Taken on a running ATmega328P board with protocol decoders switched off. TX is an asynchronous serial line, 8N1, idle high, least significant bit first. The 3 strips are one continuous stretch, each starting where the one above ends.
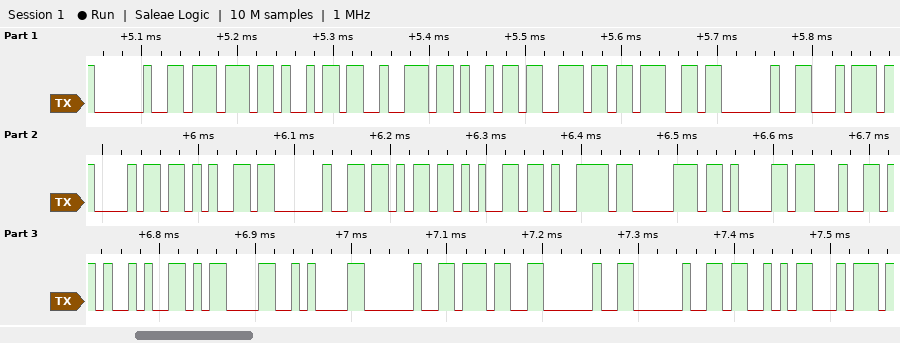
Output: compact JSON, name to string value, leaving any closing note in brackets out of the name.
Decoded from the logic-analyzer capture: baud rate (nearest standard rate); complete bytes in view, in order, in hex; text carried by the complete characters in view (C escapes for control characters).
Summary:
{"baud rate": "115200 baud", "complete bytes in view, in order, in hex": "20 77 69 72 69 6E 67 20 74 68 65 20 6B 65 79 70 61 64 29 0D 0A 20 37 20 20 53 74", "text carried by the complete characters in view": "\" wiring the keypad)\\r\\n 7  St\""}
